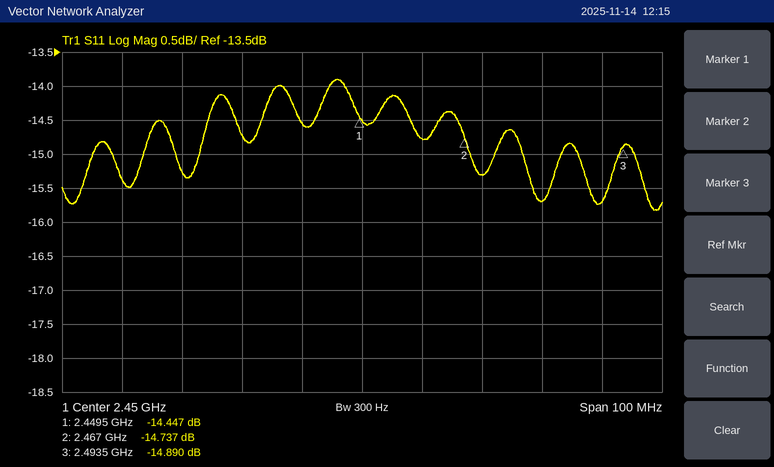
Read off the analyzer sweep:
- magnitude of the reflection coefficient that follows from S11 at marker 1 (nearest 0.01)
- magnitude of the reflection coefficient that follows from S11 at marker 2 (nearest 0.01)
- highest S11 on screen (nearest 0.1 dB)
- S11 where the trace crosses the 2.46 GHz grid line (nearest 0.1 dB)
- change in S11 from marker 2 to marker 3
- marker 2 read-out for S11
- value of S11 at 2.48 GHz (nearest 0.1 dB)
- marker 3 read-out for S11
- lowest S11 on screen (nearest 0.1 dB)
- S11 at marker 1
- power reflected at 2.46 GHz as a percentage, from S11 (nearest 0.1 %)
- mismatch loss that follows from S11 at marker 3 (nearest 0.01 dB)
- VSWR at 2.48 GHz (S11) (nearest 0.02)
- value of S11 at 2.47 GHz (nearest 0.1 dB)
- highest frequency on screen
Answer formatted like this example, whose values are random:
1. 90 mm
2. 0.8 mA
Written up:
1. 0.19
2. 0.18
3. -13.9 dB
4. -14.8 dB
5. -0.153 dB
6. -14.737 dB
7. -15.7 dB
8. -14.890 dB
9. -15.8 dB
10. -14.447 dB
11. 3.3 %
12. 0.14 dB
13. 1.40
14. -15.3 dB
15. 2.5 GHz
